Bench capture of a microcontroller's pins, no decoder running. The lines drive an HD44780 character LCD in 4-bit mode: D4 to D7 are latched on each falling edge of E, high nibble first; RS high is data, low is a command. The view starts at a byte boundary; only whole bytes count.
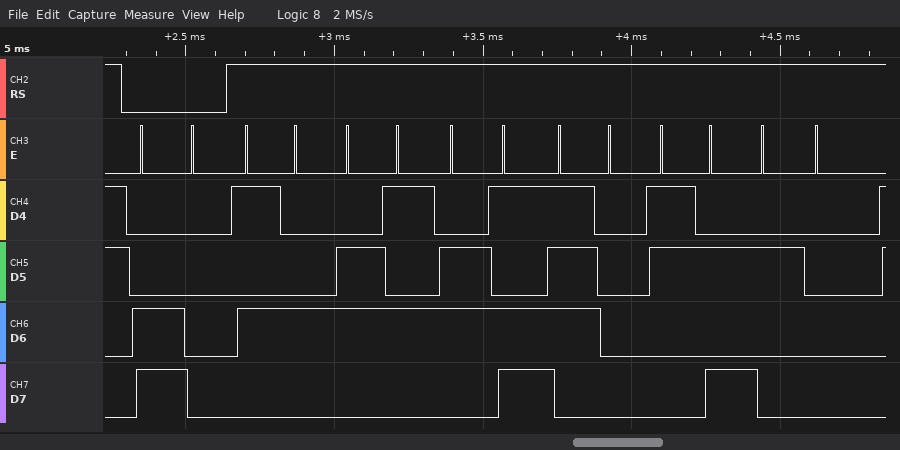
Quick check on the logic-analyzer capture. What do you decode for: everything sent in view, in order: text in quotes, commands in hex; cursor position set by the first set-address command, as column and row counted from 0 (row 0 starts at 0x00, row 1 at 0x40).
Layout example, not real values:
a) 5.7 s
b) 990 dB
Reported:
a) 0xC0 "Temp: "
b) column 0, row 1
